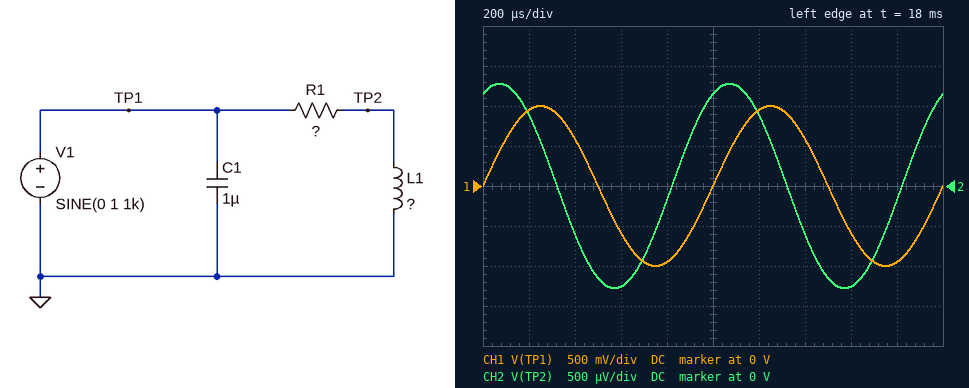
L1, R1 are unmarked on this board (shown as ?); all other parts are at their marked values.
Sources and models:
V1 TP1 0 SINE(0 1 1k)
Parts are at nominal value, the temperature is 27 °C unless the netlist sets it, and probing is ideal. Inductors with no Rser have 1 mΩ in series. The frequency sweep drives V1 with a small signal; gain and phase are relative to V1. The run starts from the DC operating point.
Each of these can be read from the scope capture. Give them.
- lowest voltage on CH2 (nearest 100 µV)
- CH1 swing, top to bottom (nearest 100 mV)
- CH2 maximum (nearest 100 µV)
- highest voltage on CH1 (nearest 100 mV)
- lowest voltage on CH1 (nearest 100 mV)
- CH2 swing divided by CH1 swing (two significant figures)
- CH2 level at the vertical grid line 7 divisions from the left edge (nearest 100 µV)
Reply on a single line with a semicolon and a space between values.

-1.3 mV; 2.0 V; 1.3 mV; 1.0 V; -1.0 V; 0.0013; -600 µV
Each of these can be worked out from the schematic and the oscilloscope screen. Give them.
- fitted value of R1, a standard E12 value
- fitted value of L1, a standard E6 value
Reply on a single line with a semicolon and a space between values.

1.8 Ω; 330 nH
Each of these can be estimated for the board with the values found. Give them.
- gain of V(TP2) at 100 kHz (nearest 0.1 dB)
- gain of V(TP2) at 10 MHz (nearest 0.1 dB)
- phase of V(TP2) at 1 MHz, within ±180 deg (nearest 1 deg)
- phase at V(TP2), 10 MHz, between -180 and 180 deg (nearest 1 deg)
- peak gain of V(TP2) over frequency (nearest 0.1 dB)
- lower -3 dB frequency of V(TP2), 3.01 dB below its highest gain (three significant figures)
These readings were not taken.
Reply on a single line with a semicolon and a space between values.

-18.8 dB; 0 dB; 41 deg; 5 deg; 0 dB; 869 kHz
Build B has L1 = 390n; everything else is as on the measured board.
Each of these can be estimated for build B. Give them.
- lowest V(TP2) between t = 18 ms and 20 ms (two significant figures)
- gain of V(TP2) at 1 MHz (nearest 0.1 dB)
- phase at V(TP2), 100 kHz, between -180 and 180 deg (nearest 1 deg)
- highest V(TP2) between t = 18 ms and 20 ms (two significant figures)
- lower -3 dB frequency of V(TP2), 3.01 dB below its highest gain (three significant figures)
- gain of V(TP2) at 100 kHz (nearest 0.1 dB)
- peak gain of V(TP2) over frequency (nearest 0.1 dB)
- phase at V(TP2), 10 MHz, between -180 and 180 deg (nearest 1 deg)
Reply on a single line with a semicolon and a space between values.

-1.5 mV; -1.9 dB; 82 deg; 1.5 mV; 735 kHz; -17.4 dB; 0 dB; 4 deg
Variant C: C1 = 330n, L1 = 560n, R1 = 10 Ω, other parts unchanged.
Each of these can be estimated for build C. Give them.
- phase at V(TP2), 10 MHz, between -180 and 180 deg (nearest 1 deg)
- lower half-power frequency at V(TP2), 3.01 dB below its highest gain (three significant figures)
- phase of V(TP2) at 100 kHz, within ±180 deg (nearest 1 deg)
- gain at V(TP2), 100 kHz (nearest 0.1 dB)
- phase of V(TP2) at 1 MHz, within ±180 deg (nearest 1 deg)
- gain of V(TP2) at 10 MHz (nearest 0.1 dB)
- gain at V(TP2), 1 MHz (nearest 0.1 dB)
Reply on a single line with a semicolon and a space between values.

16 deg; 2.84 MHz; 88 deg; -29.1 dB; 71 deg; -0.3 dB; -9.6 dB
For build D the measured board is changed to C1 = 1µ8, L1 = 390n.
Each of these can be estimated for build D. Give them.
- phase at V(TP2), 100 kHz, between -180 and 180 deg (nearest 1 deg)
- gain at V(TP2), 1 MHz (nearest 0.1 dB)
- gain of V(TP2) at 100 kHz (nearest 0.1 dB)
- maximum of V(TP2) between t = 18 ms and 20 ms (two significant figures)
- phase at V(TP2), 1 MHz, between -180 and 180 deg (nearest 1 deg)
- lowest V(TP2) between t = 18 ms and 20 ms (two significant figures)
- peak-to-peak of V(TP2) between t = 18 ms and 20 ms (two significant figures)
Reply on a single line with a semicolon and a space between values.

82 deg; -1.9 dB; -17.4 dB; 1.5 mV; 36 deg; -1.5 mV; 2.9 mV
